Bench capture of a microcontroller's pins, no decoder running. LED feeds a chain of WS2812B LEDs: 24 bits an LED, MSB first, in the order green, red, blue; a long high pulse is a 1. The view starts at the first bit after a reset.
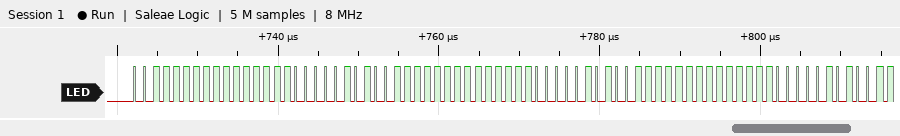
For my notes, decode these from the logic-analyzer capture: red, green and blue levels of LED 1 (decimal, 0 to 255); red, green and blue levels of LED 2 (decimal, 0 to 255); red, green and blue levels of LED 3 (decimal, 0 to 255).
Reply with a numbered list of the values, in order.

1. 255, 63, 5
2. 255, 63, 5
3. 255, 63, 5
